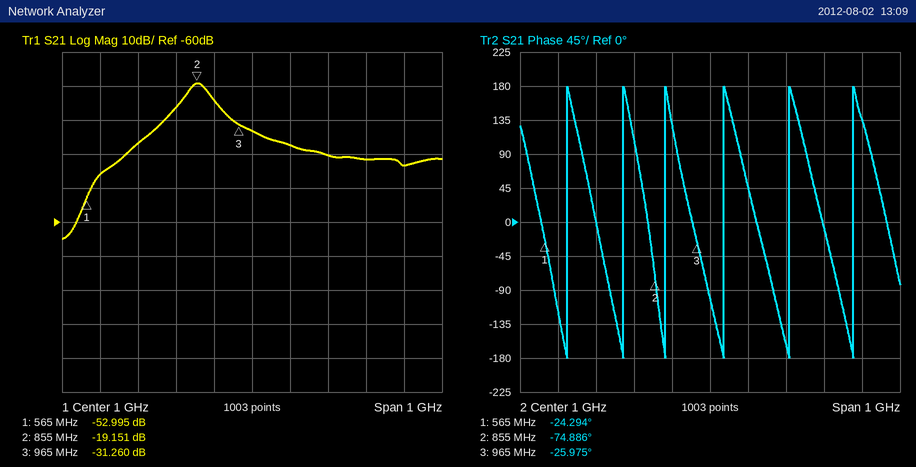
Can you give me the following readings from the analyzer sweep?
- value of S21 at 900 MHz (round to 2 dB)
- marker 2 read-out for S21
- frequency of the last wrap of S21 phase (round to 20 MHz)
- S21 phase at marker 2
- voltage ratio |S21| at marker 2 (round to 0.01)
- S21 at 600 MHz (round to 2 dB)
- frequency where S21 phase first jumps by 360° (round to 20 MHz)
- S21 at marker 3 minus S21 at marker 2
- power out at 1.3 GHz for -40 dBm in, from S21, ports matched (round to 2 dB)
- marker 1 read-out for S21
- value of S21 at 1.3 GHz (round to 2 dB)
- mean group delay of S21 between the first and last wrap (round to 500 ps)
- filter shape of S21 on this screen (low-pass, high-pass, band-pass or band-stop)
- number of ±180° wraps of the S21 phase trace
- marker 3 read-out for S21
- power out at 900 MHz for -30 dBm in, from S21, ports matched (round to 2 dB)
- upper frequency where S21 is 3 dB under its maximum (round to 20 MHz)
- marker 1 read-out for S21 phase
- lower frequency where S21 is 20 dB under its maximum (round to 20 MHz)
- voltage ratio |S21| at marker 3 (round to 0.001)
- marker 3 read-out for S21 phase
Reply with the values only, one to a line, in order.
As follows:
-24 dB
-19.151 dB
1.38 GHz
-74.886°
0.11
-46 dB
620 MHz
-12.109 dB
-82 dBm
-52.995 dB
-42 dB
6.5 ns
band-pass
6
-31.260 dB
-54 dBm
880 MHz
-24.294°
680 MHz
0.027
-25.975°
